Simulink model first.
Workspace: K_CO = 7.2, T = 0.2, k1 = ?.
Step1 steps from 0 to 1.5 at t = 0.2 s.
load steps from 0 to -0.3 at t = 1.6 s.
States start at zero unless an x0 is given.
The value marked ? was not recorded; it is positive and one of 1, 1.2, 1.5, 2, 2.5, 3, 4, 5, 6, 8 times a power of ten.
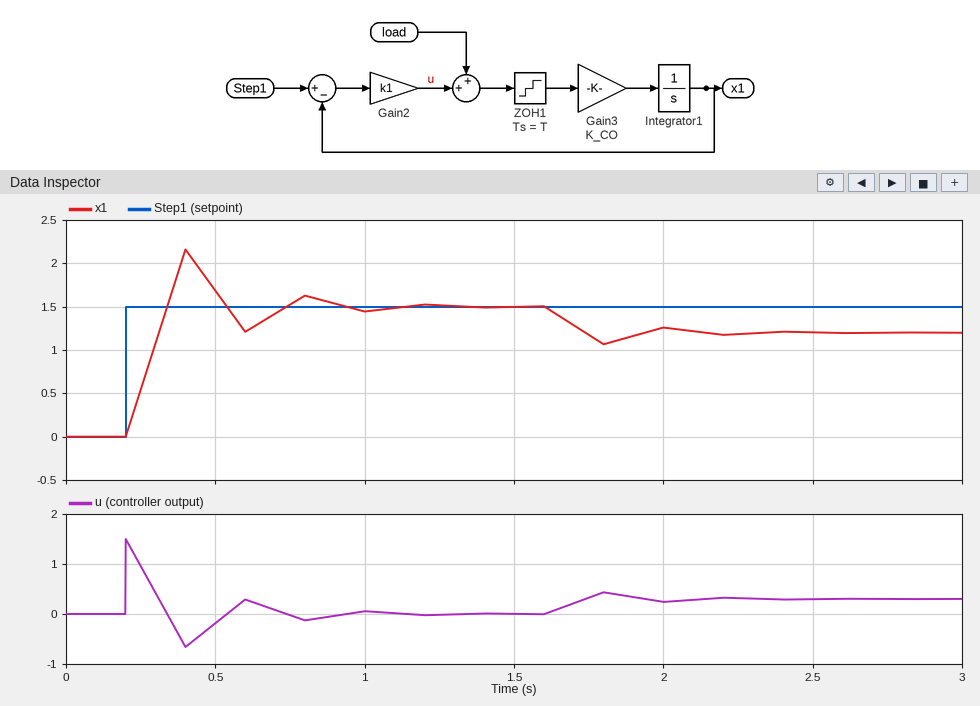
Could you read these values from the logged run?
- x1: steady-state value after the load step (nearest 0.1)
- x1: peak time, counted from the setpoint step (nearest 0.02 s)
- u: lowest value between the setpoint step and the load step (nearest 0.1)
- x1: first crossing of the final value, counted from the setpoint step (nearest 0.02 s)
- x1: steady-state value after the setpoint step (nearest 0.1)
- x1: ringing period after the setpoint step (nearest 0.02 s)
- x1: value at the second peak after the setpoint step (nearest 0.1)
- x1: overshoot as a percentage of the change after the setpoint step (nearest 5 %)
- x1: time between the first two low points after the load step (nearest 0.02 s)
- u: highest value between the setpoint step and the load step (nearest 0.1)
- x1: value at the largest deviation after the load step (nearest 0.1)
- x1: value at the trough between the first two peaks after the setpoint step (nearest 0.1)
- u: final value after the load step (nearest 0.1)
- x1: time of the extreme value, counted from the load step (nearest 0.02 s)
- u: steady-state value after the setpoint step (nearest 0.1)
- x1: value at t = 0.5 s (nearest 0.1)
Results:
1.2
0.20 s
-0.7
0.14 s
1.5
0.40 s
1.6
45 %
0.40 s
1.5
1.1
1.2
0.3
0.20 s
0.0
1.7
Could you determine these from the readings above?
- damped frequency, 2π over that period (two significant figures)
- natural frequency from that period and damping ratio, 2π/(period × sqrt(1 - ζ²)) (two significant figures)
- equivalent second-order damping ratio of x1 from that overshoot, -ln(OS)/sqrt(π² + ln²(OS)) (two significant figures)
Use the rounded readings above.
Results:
16 rad/s
16 rad/s
0.25
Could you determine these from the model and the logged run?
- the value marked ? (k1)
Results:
1
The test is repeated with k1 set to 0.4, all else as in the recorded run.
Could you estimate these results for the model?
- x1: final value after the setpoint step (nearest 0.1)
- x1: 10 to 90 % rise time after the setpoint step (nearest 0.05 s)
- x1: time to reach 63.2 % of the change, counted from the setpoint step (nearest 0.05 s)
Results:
1.5
0.50 s
0.25 s
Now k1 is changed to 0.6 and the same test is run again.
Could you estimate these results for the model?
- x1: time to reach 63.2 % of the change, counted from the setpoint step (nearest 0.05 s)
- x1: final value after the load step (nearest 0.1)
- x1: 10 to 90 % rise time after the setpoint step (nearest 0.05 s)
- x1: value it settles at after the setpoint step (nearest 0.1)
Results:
0.15 s
1.0
0.25 s
1.5
